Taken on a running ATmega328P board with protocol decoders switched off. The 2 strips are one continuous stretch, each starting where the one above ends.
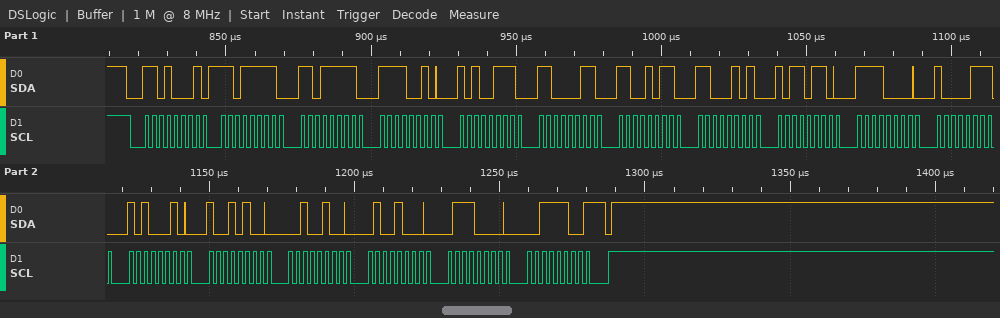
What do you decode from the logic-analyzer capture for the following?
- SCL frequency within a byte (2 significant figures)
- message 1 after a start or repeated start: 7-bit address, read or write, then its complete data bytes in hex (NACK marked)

400 kHz
0x68 read: DF DF F2 A7 C3 CB C5 B6 F0 87 A2 94 24 48 70 3C NACK
